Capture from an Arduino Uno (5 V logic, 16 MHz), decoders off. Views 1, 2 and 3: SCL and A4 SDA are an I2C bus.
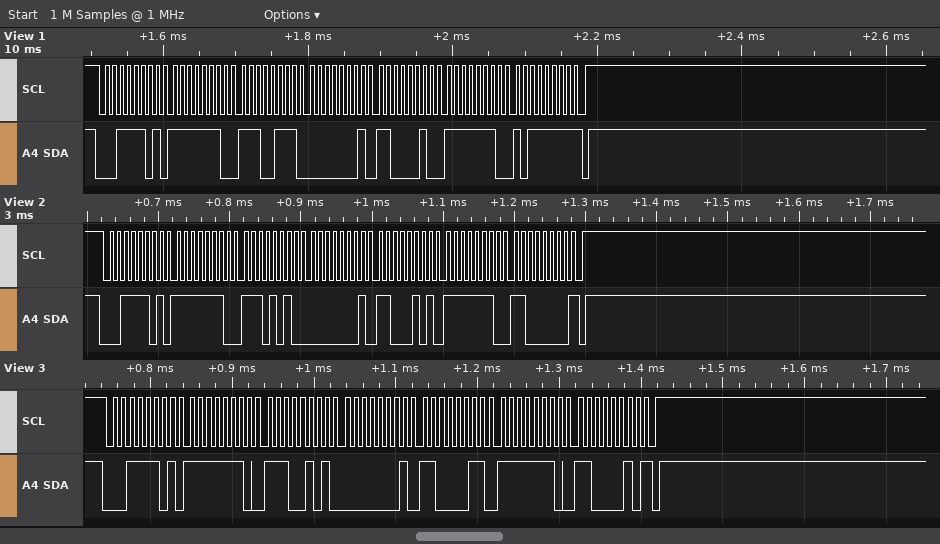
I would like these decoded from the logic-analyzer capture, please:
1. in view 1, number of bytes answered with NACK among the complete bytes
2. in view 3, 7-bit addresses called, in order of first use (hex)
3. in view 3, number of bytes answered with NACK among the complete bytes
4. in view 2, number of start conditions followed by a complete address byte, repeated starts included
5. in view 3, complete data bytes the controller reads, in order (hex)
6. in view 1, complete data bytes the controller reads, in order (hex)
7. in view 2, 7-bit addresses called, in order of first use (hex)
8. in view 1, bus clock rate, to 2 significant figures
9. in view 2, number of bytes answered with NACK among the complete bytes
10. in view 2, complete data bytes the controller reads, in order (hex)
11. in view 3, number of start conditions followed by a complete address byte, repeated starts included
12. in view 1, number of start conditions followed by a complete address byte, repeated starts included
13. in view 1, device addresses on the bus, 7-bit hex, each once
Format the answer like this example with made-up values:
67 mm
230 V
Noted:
1
0x1E
1
1
FE E5 01 C3 FE C2
FE E7 01 C2 FE BF
0x1E
100 kHz
1
FE EA 01 C5 FE C0
1
1
0x1E
